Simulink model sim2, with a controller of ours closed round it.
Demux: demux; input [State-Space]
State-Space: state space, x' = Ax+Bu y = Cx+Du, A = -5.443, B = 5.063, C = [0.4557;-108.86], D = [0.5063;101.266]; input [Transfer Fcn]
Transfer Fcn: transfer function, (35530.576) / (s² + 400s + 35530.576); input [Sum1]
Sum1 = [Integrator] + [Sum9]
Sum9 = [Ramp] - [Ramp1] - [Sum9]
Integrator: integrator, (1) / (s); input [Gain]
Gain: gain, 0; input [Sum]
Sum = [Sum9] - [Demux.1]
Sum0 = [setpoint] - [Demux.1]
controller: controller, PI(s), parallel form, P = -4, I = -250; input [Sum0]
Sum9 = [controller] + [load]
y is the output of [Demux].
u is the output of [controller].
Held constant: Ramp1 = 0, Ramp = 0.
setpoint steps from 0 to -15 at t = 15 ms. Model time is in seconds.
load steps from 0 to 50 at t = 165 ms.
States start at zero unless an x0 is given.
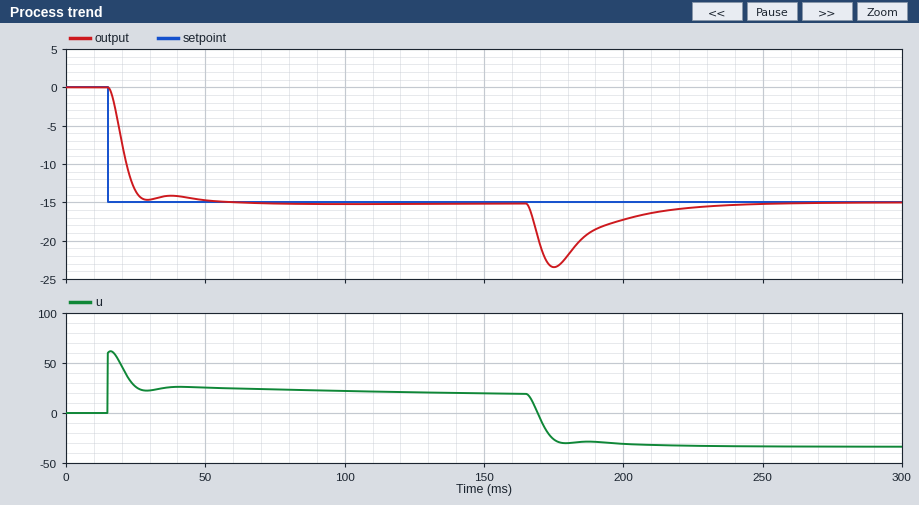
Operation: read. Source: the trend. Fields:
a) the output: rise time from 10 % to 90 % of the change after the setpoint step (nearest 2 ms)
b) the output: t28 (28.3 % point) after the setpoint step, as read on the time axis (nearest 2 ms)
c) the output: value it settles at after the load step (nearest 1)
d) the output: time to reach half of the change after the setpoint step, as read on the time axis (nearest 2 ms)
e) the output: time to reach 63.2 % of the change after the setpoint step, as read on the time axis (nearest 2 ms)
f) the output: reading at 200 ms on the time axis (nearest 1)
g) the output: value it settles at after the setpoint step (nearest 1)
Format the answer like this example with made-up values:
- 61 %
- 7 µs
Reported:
- 8 ms
- 18 ms
- -15
- 20 ms
- 22 ms
- -17
- -15
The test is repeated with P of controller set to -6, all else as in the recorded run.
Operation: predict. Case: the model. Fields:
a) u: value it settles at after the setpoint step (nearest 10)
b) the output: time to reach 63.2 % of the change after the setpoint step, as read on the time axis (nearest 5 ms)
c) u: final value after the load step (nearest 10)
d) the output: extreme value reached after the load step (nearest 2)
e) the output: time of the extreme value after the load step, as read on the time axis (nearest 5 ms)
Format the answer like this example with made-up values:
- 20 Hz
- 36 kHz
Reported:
- 20
- 20 ms
- -30
- -22
- 175 ms
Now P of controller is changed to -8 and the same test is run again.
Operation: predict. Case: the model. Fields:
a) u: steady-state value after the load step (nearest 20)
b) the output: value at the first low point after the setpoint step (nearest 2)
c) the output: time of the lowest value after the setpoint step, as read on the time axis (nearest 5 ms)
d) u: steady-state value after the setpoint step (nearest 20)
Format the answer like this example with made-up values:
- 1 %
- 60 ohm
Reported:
- -40
- -16
- 25 ms
- 20
